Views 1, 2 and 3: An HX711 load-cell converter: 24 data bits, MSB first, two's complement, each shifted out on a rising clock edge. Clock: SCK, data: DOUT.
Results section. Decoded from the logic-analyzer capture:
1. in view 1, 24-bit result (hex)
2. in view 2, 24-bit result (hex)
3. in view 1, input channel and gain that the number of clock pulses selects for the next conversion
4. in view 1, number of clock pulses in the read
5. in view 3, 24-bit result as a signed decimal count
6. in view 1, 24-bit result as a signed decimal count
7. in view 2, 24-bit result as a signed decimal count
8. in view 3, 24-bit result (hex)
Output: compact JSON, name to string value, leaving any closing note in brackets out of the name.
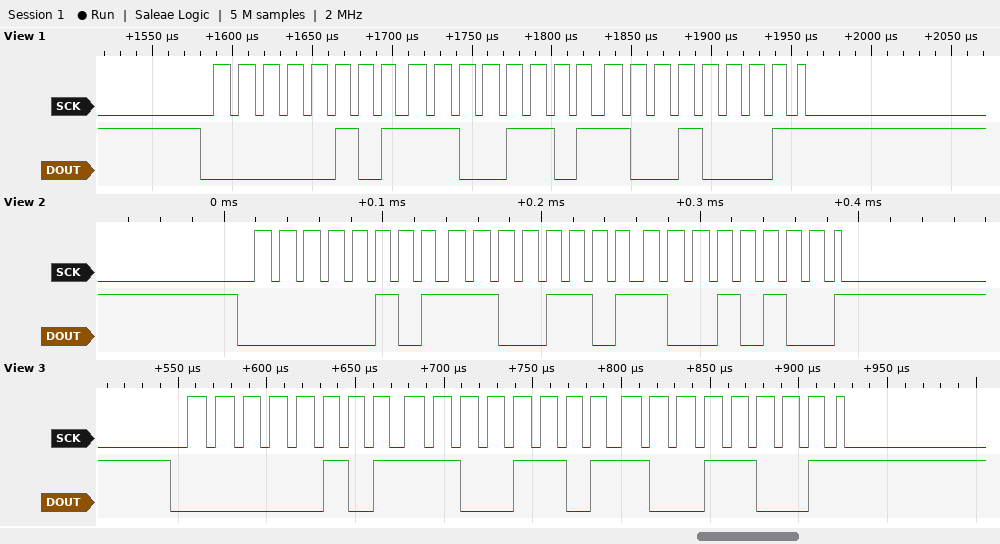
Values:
{"in view 1, 24-bit result": "0x05CD91", "in view 2, 24-bit result": "0x05CD94", "in view 1, input channel and gain that the number of clock pulses selects for the next conversion": "channel A, gain 128", "in view 1, number of clock pulses in the read": "25", "in view 3, 24-bit result as a signed decimal count": "380313", "in view 1, 24-bit result as a signed decimal count": "380305", "in view 2, 24-bit result as a signed decimal count": "380308", "in view 3, 24-bit result": "0x05CD99"}
